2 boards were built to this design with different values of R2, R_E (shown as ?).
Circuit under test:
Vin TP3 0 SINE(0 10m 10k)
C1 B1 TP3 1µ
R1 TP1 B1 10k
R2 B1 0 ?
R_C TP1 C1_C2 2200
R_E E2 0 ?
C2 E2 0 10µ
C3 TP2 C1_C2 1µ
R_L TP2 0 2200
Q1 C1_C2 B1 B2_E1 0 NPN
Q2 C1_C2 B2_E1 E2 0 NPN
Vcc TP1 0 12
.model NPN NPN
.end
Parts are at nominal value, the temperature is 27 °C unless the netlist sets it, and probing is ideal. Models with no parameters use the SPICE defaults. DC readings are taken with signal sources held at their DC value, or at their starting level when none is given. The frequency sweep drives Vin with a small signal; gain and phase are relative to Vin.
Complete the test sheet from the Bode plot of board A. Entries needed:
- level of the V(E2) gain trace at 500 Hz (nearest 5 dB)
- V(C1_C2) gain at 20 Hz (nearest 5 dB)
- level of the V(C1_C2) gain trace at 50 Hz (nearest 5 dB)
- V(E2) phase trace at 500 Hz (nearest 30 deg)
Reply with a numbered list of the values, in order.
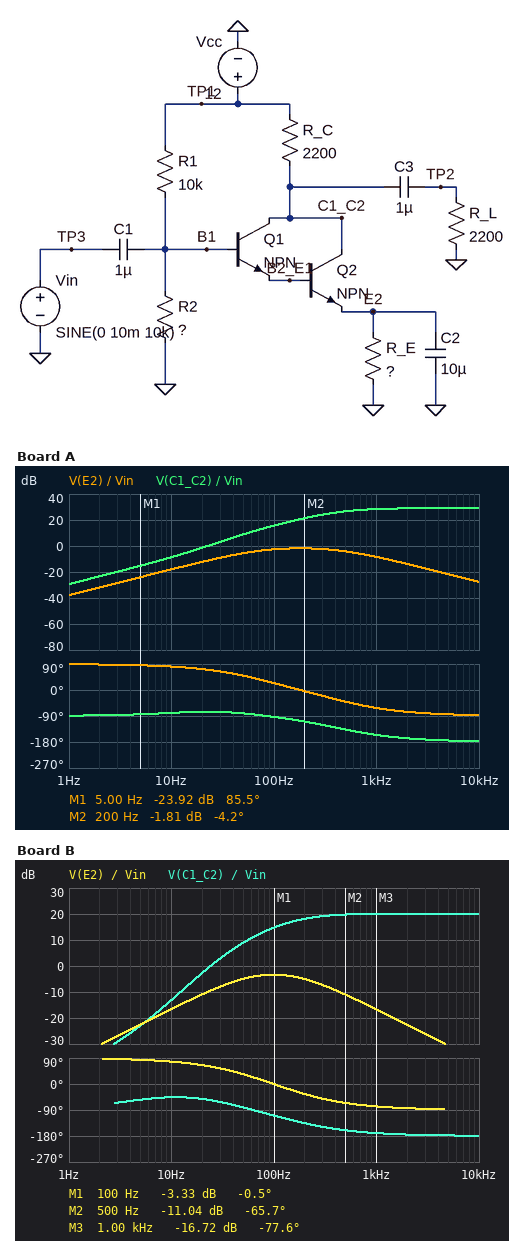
1. -5 dB
2. 0 dB
3. 10 dB
4. -30 deg
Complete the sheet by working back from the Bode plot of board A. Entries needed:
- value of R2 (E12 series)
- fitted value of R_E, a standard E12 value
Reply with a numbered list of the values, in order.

1. 2.7 kΩ
2. 820 Ω
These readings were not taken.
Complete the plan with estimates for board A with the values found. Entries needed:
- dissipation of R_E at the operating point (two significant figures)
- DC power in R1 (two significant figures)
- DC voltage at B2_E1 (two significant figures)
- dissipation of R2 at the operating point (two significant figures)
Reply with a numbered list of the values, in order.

1. 1.5 mW
2. 8.9 mW
3. 1.9 V
4. 2.4 mW
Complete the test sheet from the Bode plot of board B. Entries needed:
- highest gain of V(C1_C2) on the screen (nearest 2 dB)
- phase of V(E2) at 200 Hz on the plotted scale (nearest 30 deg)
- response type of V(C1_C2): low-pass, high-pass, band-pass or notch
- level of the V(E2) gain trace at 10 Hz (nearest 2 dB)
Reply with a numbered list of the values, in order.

1. 20 dB
2. -30 deg
3. high-pass
4. -16 dB
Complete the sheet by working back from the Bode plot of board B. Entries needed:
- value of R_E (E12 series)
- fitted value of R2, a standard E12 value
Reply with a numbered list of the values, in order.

1. 3.3 kΩ
2. 3.3 kΩ
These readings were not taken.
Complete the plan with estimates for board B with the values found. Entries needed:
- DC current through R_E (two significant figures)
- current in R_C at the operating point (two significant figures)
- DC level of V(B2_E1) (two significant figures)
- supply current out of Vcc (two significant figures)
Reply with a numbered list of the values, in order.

1. 480 µA
2. 480 µA
3. 2.3 V
4. 1.4 mA
